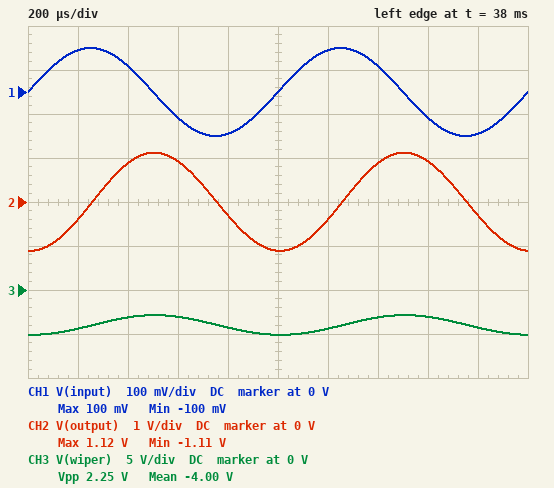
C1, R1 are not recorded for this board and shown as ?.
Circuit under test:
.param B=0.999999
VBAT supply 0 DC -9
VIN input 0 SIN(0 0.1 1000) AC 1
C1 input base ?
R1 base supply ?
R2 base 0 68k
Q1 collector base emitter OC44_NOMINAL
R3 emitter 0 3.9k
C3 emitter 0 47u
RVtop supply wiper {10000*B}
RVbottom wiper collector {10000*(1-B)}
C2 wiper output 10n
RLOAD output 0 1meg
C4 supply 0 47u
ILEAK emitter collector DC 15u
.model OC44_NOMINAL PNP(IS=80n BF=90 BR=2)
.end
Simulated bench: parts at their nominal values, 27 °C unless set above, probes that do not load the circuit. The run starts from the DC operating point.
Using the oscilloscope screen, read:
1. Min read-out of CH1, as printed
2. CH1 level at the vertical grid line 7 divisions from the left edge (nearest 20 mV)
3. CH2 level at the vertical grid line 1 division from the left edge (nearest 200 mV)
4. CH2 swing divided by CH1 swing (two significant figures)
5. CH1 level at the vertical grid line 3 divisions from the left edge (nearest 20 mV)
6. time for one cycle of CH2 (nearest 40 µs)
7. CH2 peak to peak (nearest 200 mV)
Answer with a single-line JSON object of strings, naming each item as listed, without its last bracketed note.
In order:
{"Min read-out of CH1, as printed": "-100 mV", "CH1 level at the vertical grid line 7 divisions from the left edge": "60 mV", "CH2 level at the vertical grid line 1 division from the left edge": "-400 mV", "CH2 swing divided by CH1 swing": "11", "CH1 level at the vertical grid line 3 divisions from the left edge": "-60 mV", "time for one cycle of CH2": "1.00 ms", "CH2 peak to peak": "2.2 V"}
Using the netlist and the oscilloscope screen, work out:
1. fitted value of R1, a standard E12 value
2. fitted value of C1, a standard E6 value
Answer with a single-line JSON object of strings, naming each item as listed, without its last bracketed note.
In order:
{"fitted value of R1, a standard E12 value": "180 kΩ", "fitted value of C1, a standard E6 value": "2.2 nF"}
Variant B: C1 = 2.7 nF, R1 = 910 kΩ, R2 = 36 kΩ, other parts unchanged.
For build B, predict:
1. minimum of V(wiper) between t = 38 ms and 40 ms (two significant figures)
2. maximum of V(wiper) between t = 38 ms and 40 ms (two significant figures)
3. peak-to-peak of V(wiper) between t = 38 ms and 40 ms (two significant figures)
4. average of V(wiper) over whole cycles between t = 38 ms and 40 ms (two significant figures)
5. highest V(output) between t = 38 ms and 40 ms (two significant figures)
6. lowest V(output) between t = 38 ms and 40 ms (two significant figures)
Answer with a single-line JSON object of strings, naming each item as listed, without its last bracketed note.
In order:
{"minimum of V(wiper) between t = 38 ms and 40 ms": "-8.8 V", "maximum of V(wiper) between t = 38 ms and 40 ms": "-8.0 V", "peak-to-peak of V(wiper) between t = 38 ms and 40 ms": "840 mV", "average of V(wiper) over whole cycles between t = 38 ms and 40 ms": "-8.5 V", "highest V(output) between t = 38 ms and 40 ms": "530 mV", "lowest V(output) between t = 38 ms and 40 ms": "-320 mV"}
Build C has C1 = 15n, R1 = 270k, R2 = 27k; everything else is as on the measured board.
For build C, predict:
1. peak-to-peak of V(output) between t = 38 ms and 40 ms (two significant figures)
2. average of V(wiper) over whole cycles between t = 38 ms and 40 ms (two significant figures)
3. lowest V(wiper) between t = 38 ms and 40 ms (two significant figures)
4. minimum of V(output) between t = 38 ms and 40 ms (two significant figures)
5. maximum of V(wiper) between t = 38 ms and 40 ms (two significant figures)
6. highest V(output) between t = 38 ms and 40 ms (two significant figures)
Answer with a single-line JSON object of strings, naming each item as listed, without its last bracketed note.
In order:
{"peak-to-peak of V(output) between t = 38 ms and 40 ms": "5.7 V", "average of V(wiper) over whole cycles between t = 38 ms and 40 ms": "-7.3 V", "lowest V(wiper) between t = 38 ms and 40 ms": "-8.8 V", "minimum of V(output) between t = 38 ms and 40 ms": "-1.6 V", "maximum of V(wiper) between t = 38 ms and 40 ms": "-3.2 V", "highest V(output) between t = 38 ms and 40 ms": "4.1 V"}
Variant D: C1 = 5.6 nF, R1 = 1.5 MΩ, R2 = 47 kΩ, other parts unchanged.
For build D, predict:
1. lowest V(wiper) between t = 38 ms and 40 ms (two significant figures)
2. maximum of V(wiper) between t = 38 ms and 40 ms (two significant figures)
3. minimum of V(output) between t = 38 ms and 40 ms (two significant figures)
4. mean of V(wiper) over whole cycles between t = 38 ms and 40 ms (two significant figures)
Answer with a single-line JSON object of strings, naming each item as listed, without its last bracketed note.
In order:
{"lowest V(wiper) between t = 38 ms and 40 ms": "-8.8 V", "maximum of V(wiper) between t = 38 ms and 40 ms": "-7.6 V", "minimum of V(output) between t = 38 ms and 40 ms": "-340 mV", "mean of V(wiper) over whole cycles between t = 38 ms and 40 ms": "-8.5 V"}
